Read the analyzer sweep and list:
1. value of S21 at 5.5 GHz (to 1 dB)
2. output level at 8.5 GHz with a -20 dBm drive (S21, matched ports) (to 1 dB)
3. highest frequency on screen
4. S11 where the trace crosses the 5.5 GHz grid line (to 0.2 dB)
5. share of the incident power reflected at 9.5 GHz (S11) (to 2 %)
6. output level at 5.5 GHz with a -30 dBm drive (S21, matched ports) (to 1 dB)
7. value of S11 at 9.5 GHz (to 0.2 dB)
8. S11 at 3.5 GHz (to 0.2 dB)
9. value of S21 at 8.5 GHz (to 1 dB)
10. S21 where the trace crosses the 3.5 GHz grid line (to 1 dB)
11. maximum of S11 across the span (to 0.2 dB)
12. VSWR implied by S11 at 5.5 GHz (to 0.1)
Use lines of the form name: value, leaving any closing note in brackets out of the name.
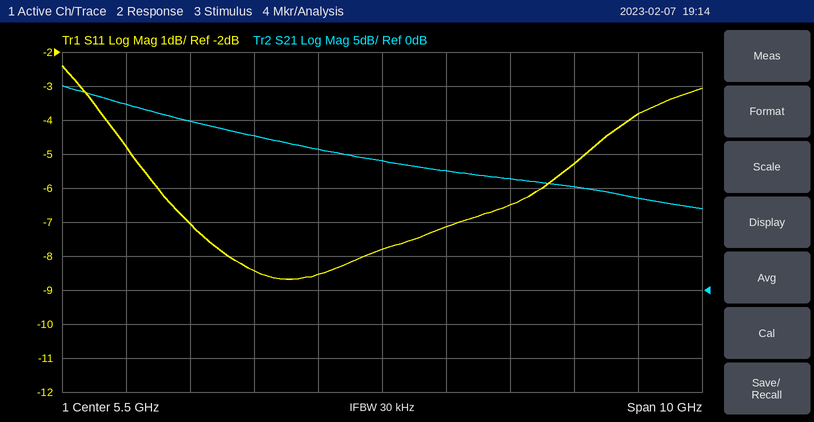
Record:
value of S21 at 5.5 GHz: 19 dB
output level at 8.5 GHz with a -20 dBm drive (S21, matched ports): -5 dBm
highest frequency on screen: 10.5 GHz
S11 where the trace crosses the 5.5 GHz grid line: -7.8 dB
share of the incident power reflected at 9.5 GHz (S11): 42 %
output level at 5.5 GHz with a -30 dBm drive (S21, matched ports): -11 dBm
value of S11 at 9.5 GHz: -3.8 dB
S11 at 3.5 GHz: -8.4 dB
value of S21 at 8.5 GHz: 15 dB
S21 where the trace crosses the 3.5 GHz grid line: 23 dB
maximum of S11 across the span: -2.4 dB
VSWR implied by S11 at 5.5 GHz: 2.4
